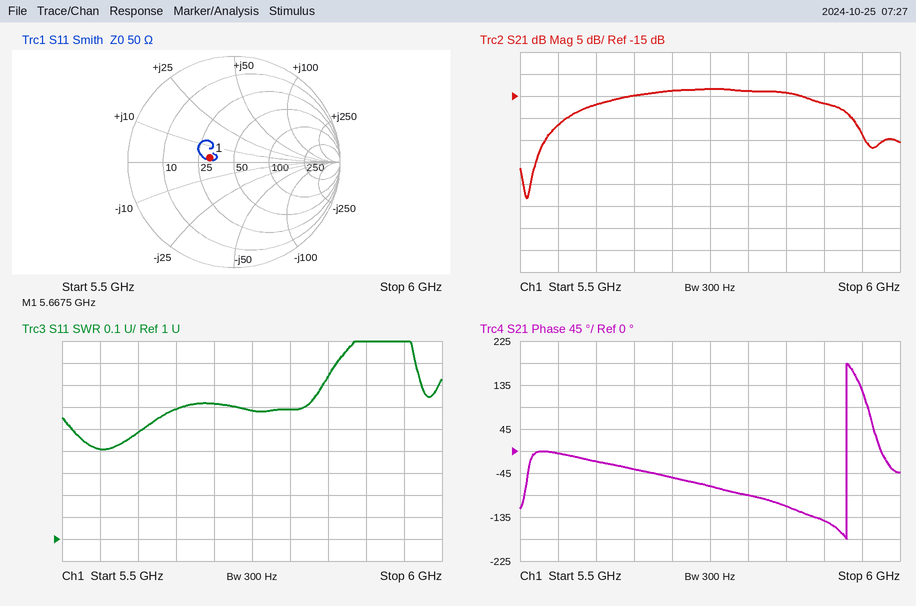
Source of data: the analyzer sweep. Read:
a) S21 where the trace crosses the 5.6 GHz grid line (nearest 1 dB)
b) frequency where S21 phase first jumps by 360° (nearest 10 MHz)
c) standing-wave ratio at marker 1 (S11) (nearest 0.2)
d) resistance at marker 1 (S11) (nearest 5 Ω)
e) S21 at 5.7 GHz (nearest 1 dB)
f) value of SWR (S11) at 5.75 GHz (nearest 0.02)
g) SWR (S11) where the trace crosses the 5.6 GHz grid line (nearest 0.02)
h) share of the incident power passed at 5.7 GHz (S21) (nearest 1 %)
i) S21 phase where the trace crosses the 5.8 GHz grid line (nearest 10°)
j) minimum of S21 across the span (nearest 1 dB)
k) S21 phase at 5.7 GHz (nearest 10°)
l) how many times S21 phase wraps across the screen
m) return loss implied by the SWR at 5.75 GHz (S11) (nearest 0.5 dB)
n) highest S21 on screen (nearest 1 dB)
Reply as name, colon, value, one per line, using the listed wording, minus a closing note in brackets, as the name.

S21 where the trace crosses the 5.6 GHz grid line: -17 dB
frequency where S21 phase first jumps by 360°: 5.93 GHz
standing-wave ratio at marker 1 (S11): 1.6
resistance at marker 1 (S11): 30 Ω
S21 at 5.7 GHz: -14 dB
value of SWR (S11) at 5.75 GHz: 1.58
SWR (S11) where the trace crosses the 5.6 GHz grid line: 1.48
share of the incident power passed at 5.7 GHz (S21): 4 %
S21 phase where the trace crosses the 5.8 GHz grid line: -90°
minimum of S21 across the span: -38 dB
S21 phase at 5.7 GHz: -50°
how many times S21 phase wraps across the screen: 1
return loss implied by the SWR at 5.75 GHz (S11): 13.0 dB
highest S21 on screen: -13 dB
